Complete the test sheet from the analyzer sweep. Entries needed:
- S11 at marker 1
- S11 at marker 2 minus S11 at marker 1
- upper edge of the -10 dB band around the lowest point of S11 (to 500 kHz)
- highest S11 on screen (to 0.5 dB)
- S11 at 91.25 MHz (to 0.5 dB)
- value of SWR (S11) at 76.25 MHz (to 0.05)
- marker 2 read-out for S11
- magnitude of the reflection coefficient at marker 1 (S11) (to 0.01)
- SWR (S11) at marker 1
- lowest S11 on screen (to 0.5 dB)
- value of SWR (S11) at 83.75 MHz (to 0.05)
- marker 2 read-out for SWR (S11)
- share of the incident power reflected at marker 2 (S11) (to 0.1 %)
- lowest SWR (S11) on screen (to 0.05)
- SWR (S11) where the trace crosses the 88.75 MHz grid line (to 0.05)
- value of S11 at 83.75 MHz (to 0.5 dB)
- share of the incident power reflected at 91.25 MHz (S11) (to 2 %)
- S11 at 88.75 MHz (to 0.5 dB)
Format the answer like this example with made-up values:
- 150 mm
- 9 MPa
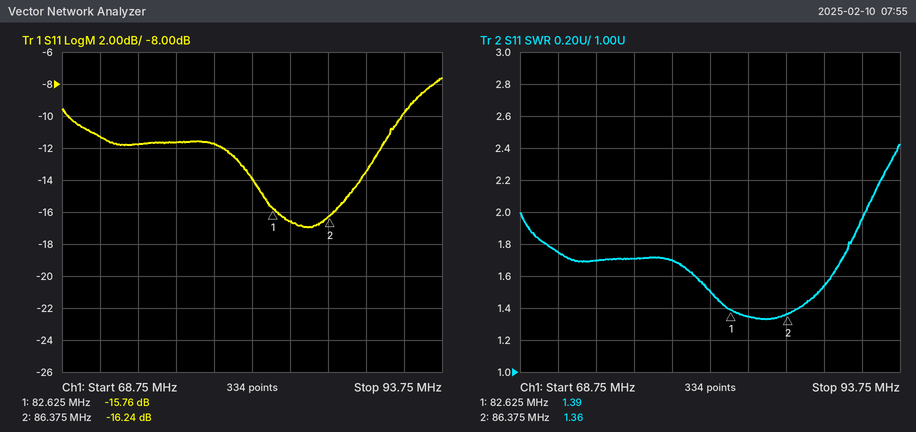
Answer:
- -15.76 dB
- -0.48 dB
- 91.0 MHz
- -7.5 dB
- -10.0 dB
- 1.70
- -16.24 dB
- 0.16
- 1.39
- -17.0 dB
- 1.35
- 1.36
- 2.4 %
- 1.35
- 1.55
- -16.5 dB
- 10 %
- -13.5 dB
